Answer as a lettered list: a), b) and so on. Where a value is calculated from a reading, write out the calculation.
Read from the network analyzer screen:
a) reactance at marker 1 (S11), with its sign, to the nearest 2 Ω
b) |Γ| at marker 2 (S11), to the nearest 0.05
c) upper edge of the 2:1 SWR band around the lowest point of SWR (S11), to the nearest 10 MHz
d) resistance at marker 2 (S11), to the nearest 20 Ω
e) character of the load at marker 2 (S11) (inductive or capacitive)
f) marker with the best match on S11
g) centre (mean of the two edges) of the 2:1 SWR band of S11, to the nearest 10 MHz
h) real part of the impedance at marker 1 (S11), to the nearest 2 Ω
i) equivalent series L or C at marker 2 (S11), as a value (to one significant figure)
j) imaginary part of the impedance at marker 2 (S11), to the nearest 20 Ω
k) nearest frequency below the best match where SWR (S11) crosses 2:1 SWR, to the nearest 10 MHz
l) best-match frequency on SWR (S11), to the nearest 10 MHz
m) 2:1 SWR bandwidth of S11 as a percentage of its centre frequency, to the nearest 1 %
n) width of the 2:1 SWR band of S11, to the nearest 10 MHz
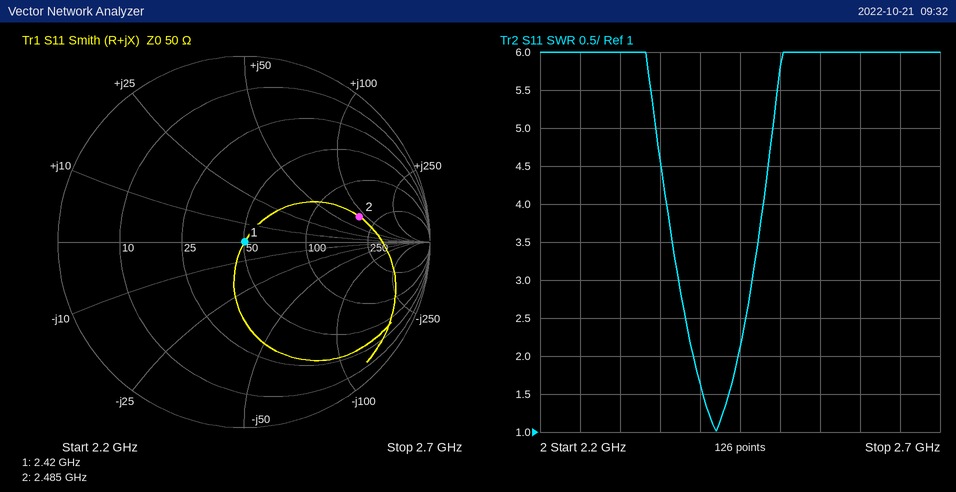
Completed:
a) 0 Ω
b) 0.65
c) 2.45 GHz
d) 180 Ω
e) inductive
f) marker 1
g) 2.42 GHz
h) 50 Ω
i) L = 80 Ω/(2π × 2.485 GHz) ≈ 5 nH
j) +80 Ω
k) 2.39 GHz
l) 2.42 GHz
m) 60 MHz / 2.42 GHz ≈ 2 %
n) 2.45 GHz − 2.39 GHz = 60 MHz
